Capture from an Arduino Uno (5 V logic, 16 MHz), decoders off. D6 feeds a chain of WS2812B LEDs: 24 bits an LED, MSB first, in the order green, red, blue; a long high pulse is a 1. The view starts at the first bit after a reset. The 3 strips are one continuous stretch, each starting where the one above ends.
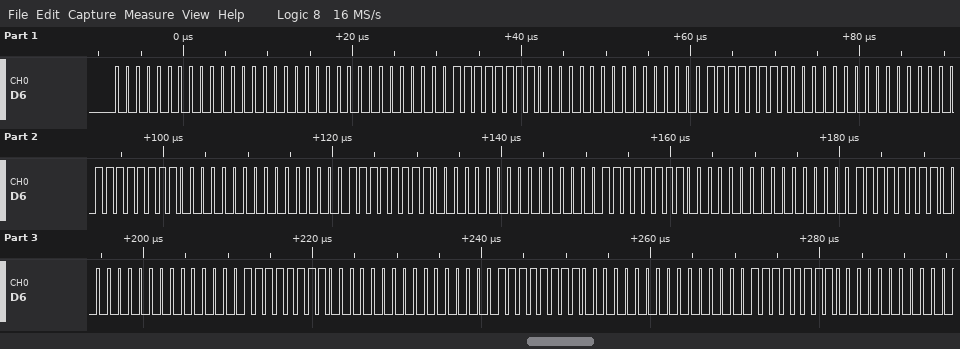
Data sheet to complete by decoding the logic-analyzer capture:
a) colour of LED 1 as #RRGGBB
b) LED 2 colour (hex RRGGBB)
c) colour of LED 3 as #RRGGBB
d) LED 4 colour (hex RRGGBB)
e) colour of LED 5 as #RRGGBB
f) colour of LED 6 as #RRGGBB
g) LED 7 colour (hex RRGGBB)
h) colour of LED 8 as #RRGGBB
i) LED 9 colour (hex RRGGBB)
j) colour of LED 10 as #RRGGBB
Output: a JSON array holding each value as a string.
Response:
["#000000", "#FF0000", "#FF0000", "#FF0000", "#FF0000", "#FF0000", "#FF0000", "#FF0000", "#FF0000", "#FF0000"]
